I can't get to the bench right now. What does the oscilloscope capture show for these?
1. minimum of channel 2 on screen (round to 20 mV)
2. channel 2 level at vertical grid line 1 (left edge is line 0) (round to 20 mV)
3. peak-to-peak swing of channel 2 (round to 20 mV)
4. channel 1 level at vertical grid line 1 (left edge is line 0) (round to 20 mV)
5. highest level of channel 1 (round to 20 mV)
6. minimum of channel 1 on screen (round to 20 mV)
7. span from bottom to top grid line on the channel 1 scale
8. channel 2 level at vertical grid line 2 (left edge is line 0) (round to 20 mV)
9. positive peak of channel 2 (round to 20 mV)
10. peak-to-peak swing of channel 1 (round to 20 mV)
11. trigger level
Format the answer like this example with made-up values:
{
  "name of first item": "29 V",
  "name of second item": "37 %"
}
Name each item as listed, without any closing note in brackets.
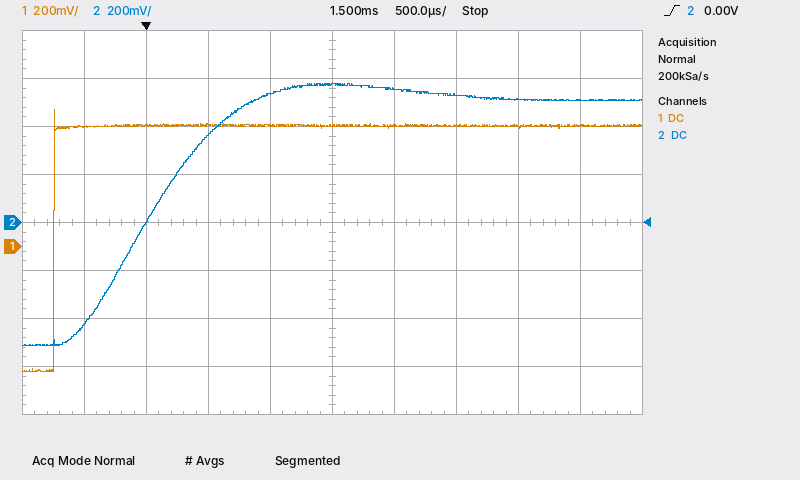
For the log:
{
  "minimum of channel 2 on screen": "-520 mV",
  "channel 2 level at vertical grid line 1 (left edge is line 0)": "-420 mV",
  "peak-to-peak swing of channel 2": "1.10 V",
  "channel 1 level at vertical grid line 1 (left edge is line 0)": "500 mV",
  "highest level of channel 1": "580 mV",
  "minimum of channel 1 on screen": "-520 mV",
  "span from bottom to top grid line on the channel 1 scale": "1.6 V",
  "channel 2 level at vertical grid line 2 (left edge is line 0)": "0 mV",
  "positive peak of channel 2": "580 mV",
  "peak-to-peak swing of channel 1": "1.10 V",
  "trigger level": "0.00 V"
}
